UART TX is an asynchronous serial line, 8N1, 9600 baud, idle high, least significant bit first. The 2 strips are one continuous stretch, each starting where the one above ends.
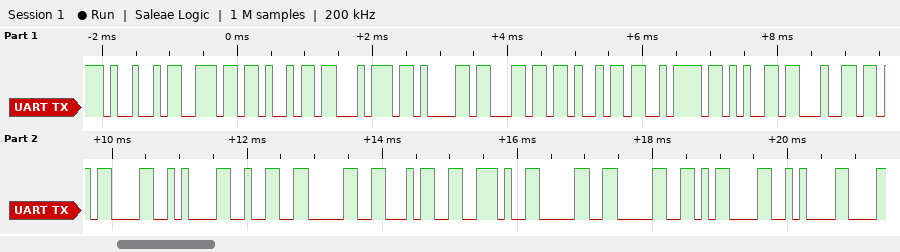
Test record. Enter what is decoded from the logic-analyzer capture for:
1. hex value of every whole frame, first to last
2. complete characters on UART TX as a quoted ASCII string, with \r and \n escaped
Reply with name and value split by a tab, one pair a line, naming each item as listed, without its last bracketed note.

hex value of every whole frame, first to last	49 6E 69 74 61 6C 69 7A 65 64 0D 0A 32 30 34 2E 30 30 0D 0A
complete characters on UART TX as a quoted ASCII string, with \r and \n escaped	"Initalized\r\n204.00\r\n"
